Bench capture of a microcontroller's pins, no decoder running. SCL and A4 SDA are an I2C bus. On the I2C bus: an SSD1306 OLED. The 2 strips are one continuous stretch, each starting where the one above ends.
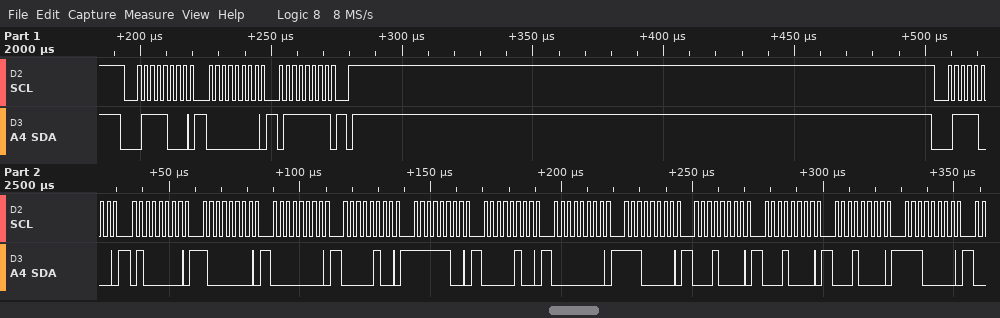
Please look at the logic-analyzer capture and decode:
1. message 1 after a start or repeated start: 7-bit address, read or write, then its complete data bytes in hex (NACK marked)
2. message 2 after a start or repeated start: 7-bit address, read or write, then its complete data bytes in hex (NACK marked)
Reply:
0x3C write: 00 7F
0x3C write: 40 80 00 04 FC 04 00 E0 10 10 10 E0
